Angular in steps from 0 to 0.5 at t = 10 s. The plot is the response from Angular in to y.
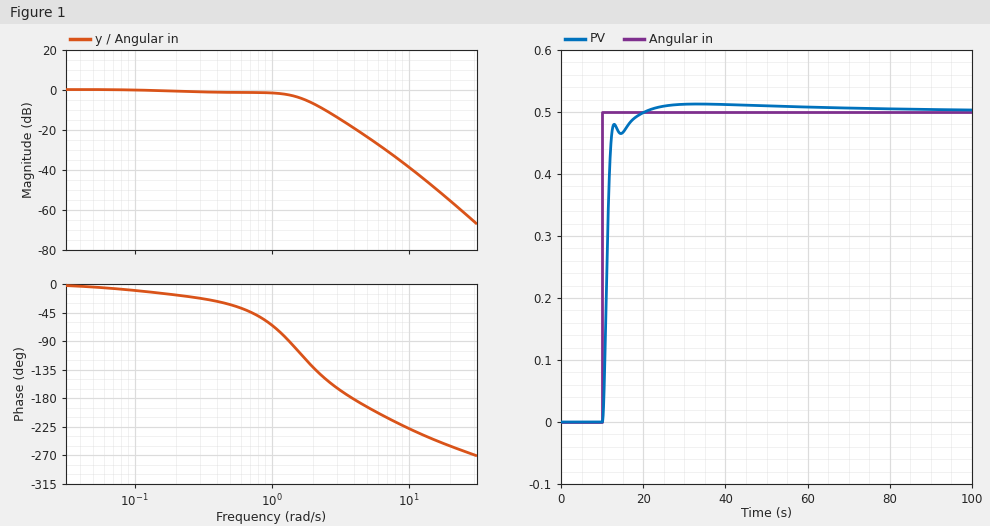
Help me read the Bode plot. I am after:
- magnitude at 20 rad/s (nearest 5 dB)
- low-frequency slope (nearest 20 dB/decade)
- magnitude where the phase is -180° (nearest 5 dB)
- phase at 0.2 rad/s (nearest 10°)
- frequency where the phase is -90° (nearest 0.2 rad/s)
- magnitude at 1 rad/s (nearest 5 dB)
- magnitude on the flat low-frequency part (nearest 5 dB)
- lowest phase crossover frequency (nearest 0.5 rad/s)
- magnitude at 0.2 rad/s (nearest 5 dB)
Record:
-55 dB
0 dB/decade
-20 dB
-20°
1.4 rad/s
0 dB
0 dB
4.0 rad/s
0 dB
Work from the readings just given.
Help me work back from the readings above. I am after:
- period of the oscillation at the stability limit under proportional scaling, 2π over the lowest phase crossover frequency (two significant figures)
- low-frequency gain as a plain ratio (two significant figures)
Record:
1.6 s
1.0
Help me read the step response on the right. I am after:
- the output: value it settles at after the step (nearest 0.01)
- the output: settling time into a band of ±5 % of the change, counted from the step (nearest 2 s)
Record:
0.50
6 s
